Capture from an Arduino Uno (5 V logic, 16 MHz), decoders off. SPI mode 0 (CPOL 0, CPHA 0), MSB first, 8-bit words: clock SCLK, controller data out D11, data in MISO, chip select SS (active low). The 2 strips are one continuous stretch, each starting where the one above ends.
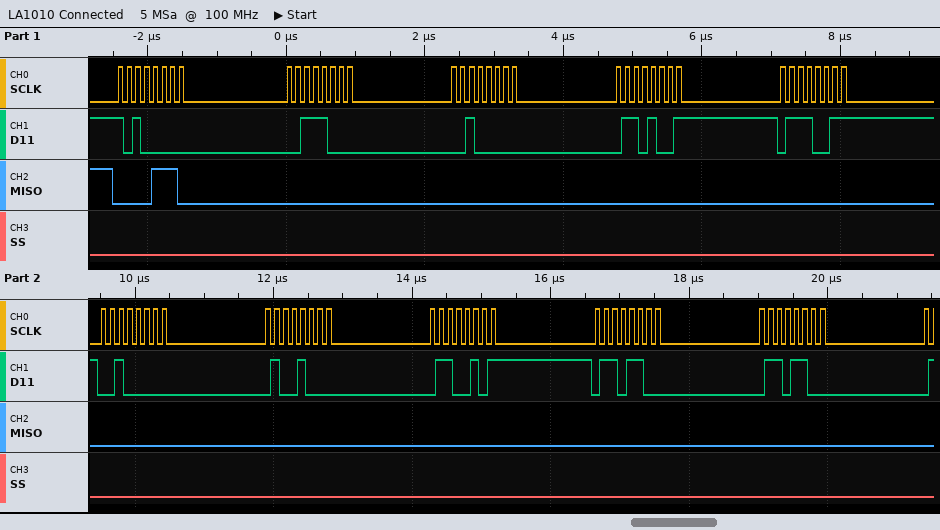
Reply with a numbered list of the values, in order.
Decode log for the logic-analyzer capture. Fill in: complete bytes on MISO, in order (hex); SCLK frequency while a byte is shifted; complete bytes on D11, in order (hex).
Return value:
1. 0x0E 0x00 0x00 0x00 0x00 0x00 0x00 0x00 0x00 0x00
2. 8 MHz
3. 0xA0 0x38 0x20 0x69 0x73 0x20 0x48 0x65 0x6C 0x6C
